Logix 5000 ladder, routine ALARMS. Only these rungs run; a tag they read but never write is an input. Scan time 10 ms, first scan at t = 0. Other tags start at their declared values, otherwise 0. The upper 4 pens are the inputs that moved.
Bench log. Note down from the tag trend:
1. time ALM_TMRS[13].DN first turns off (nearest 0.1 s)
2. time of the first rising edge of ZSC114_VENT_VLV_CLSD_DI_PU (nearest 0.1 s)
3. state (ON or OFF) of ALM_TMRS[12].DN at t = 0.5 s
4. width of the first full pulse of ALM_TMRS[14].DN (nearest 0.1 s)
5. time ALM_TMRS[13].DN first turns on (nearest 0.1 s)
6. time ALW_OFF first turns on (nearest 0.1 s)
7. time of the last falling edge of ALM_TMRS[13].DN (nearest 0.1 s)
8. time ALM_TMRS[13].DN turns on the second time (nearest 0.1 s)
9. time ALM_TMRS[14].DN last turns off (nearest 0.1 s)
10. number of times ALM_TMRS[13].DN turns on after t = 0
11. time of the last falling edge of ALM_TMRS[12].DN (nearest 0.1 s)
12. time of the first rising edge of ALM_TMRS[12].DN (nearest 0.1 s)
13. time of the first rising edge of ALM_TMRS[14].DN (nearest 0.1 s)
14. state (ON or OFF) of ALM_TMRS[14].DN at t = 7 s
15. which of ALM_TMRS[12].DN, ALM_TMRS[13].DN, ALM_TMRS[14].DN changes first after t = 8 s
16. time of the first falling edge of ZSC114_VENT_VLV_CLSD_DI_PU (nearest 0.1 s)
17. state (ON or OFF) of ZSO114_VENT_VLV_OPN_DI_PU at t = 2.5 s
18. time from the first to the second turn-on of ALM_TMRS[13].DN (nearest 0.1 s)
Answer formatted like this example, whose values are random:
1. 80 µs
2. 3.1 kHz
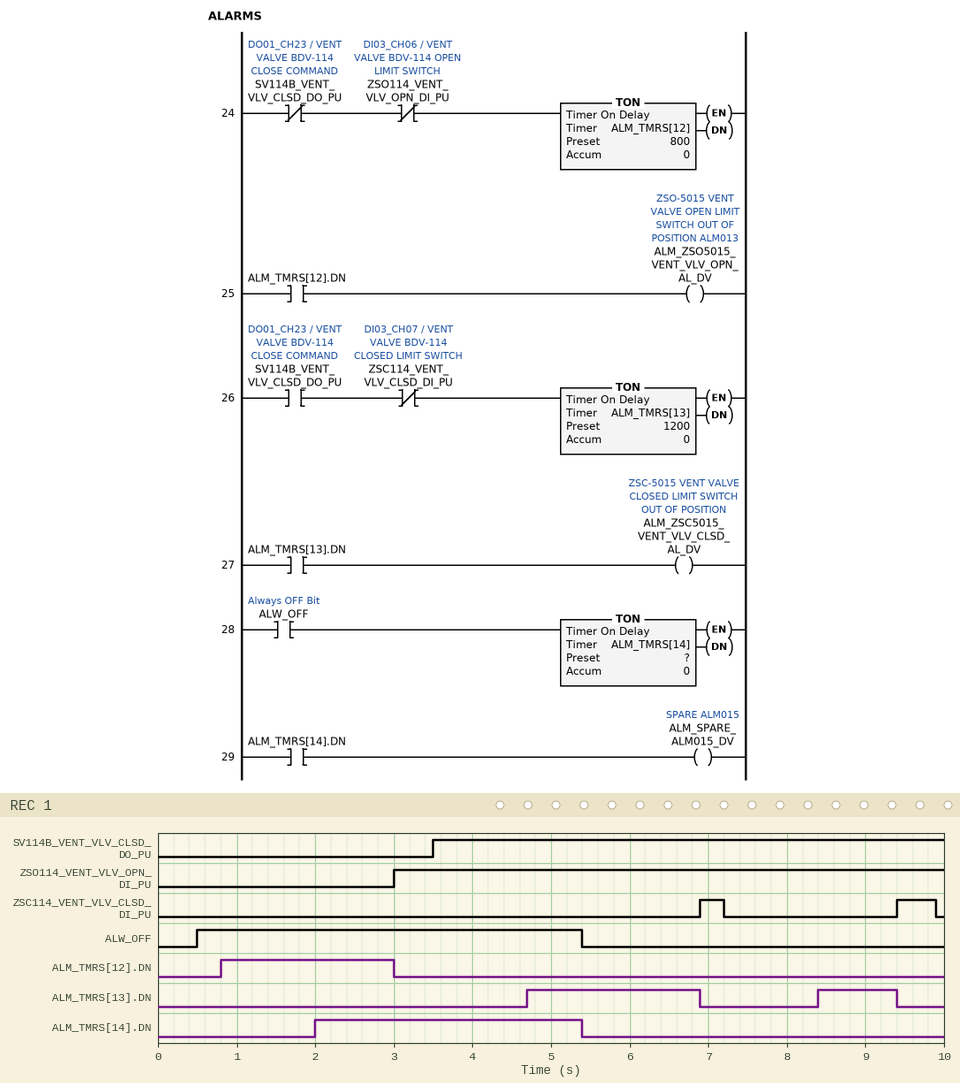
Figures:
1. 6.9 s
2. 6.9 s
3. OFF
4. 3.4 s
5. 4.7 s
6. 0.5 s
7. 9.4 s
8. 8.4 s
9. 5.4 s
10. 2
11. 3.0 s
12. 0.8 s
13. 2.0 s
14. OFF
15. ALM_TMRS[13].DN
16. 7.2 s
17. OFF
18. 3.7 s
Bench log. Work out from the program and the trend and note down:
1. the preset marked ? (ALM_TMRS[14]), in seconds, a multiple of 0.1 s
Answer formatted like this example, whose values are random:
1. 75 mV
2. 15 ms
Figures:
1. 1.5 s
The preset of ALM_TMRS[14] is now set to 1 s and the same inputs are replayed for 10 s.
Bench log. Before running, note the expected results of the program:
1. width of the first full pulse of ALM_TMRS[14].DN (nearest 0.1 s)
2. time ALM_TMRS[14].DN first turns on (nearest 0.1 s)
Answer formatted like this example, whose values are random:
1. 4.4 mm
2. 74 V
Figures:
1. 3.9 s
2. 1.5 s
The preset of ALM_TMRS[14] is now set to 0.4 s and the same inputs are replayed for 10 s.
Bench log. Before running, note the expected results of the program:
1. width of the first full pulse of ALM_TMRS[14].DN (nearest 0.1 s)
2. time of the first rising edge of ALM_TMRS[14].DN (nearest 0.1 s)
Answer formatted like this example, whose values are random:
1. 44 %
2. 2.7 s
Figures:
1. 4.5 s
2. 0.9 s
